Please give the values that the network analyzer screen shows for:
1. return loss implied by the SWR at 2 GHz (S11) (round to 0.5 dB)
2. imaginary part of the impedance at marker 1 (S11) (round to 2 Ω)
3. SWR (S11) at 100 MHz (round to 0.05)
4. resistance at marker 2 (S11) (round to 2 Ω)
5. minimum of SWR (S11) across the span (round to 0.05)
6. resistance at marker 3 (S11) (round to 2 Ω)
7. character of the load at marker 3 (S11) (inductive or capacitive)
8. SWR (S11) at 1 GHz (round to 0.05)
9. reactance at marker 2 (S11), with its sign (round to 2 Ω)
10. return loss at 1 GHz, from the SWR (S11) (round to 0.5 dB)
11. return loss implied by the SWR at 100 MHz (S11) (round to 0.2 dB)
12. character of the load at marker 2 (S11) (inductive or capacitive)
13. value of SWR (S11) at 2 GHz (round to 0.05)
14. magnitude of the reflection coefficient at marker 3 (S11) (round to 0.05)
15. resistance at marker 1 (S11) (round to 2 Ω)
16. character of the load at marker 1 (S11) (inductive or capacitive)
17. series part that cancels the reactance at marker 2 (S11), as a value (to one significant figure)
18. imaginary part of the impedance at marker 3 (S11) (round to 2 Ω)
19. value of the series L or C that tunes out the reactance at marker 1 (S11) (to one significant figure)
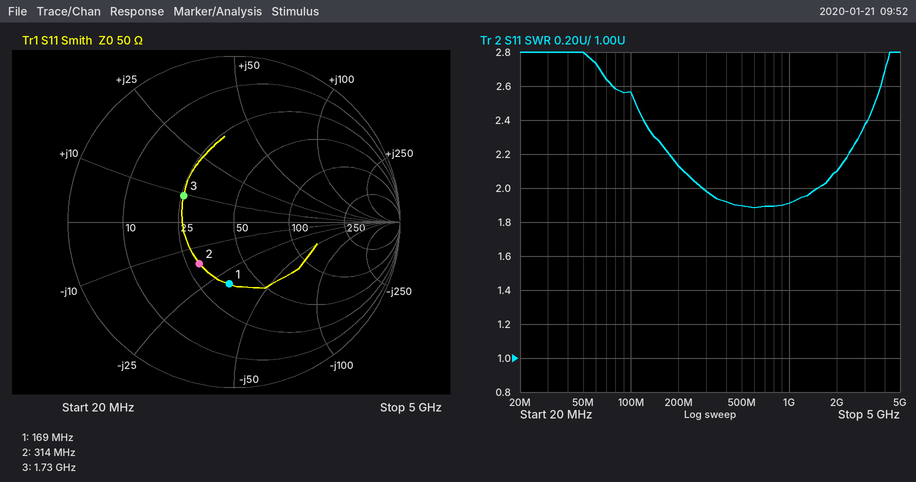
9.0 dB
-32 Ω
2.55
30 Ω
1.90
26 Ω
inductive
1.90
-16 Ω
10.0 dB
7.2 dB
capacitive
2.10
0.35
36 Ω
capacitive
8 nH
+10 Ω
30 nH
